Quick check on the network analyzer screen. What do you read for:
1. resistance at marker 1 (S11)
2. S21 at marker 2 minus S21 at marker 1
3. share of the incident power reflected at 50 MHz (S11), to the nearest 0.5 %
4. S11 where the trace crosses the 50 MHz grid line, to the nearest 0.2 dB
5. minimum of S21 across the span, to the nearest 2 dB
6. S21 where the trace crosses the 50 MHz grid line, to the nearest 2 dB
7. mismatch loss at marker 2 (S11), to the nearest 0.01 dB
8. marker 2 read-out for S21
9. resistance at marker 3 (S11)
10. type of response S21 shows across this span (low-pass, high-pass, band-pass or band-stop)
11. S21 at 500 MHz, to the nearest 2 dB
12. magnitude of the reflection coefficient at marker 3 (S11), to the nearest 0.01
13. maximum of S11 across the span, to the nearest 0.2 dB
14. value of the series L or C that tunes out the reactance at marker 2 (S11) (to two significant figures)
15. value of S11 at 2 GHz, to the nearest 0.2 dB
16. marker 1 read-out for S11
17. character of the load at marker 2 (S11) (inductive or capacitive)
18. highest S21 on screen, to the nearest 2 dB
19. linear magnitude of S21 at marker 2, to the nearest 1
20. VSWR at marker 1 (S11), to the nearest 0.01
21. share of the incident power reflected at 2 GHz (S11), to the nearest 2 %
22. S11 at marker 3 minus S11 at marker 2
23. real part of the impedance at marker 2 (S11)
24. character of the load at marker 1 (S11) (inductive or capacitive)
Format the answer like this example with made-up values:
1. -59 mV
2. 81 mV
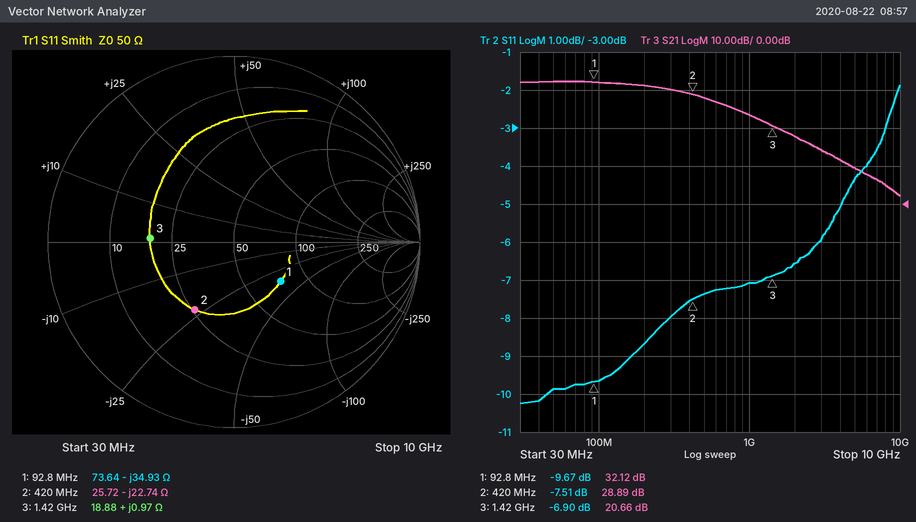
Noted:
1. 73.64 Ω
2. -3.23 dB
3. 10.5 %
4. -9.8 dB
5. 2 dB
6. 32 dB
7. 0.85 dB
8. 28.89 dB
9. 18.88 Ω
10. low-pass
11. 28 dB
12. 0.45
13. -1.8 dB
14. 8.6 nH
15. -6.6 dB
16. -9.67 dB
17. capacitive
18. 32 dB
19. 28
20. 1.98
21. 22 %
22. 0.61 dB
23. 25.72 Ω
24. capacitive
